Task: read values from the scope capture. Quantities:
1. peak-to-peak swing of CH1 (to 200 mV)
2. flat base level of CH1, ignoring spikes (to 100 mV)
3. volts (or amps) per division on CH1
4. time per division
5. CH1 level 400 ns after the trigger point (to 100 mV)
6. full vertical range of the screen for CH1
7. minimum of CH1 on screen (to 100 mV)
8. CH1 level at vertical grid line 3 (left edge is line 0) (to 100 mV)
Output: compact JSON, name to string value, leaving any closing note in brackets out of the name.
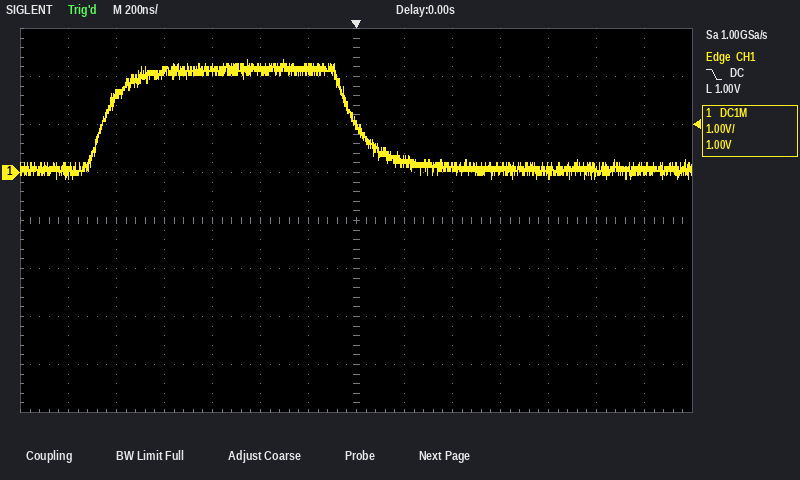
{"peak-to-peak swing of CH1": "2.4 V", "flat base level of CH1, ignoring spikes": "100 mV", "volts (or amps) per division on CH1": "1 V", "time per division": "200 ns", "CH1 level 400 ns after the trigger point": "100 mV", "full vertical range of the screen for CH1": "8 V", "minimum of CH1 on screen": "-100 mV", "CH1 level at vertical grid line 3 (left edge is line 0)": "2.1 V"}
